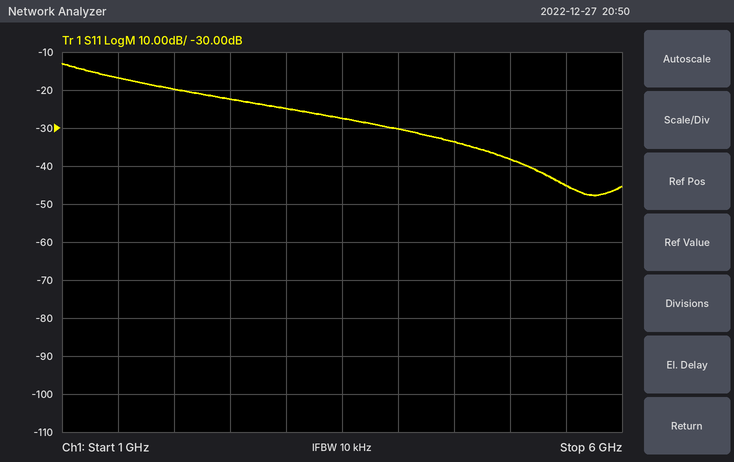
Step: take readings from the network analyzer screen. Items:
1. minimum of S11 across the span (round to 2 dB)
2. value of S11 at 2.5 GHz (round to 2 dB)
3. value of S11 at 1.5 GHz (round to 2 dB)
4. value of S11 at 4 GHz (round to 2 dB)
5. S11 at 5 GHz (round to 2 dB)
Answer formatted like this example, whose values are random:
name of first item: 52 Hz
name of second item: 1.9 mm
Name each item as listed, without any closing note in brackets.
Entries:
minimum of S11 across the span: -48 dB
value of S11 at 2.5 GHz: -22 dB
value of S11 at 1.5 GHz: -16 dB
value of S11 at 4 GHz: -30 dB
S11 at 5 GHz: -38 dB
